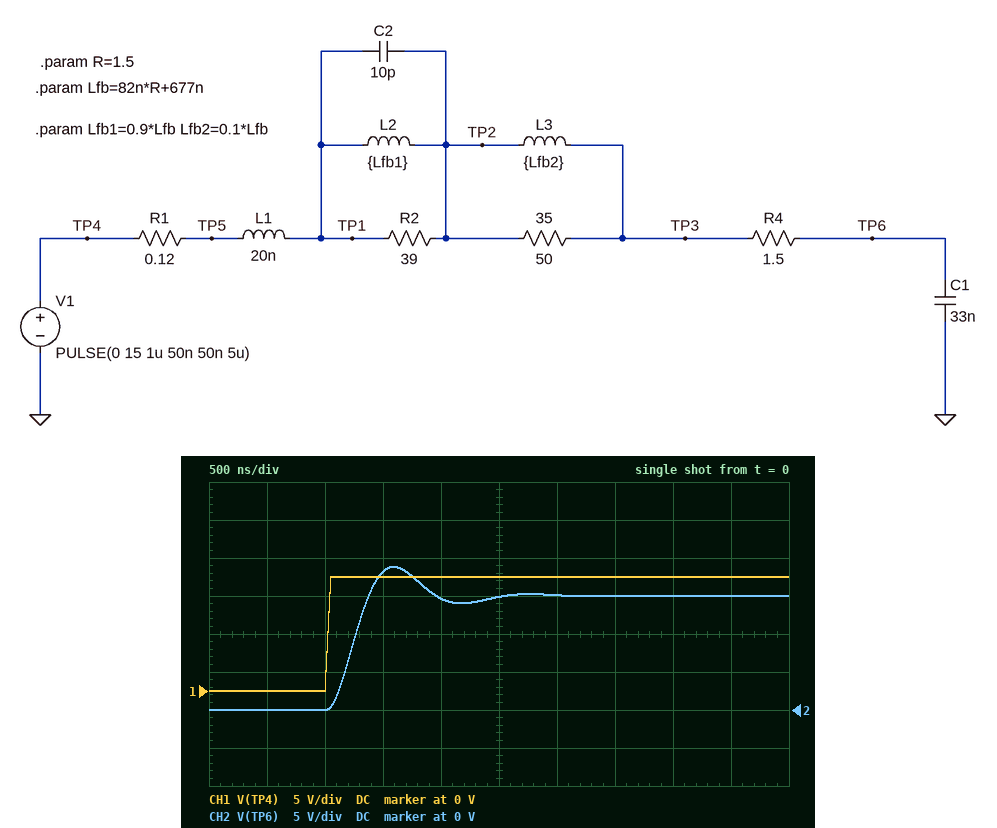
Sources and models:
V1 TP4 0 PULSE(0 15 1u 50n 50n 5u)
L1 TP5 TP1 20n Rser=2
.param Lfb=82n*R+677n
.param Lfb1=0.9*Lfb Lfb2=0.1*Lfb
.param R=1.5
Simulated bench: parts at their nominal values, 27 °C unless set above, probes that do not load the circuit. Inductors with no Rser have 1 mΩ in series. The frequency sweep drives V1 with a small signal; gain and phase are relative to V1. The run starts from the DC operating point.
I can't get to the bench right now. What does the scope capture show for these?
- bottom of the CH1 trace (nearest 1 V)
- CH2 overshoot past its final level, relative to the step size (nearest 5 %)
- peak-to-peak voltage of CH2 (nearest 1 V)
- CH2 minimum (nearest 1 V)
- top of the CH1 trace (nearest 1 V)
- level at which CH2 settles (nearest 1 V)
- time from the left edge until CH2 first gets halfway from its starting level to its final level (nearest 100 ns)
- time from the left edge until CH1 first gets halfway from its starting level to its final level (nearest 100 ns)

0 V
25 %
19 V
0 V
15 V
15 V
1.2 µs
1.0 µs
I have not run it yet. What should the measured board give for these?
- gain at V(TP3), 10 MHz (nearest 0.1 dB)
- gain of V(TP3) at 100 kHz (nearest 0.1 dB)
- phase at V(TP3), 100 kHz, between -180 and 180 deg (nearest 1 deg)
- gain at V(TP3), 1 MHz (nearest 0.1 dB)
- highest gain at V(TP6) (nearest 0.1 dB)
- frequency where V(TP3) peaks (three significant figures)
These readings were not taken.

-27.4 dB
0.1 dB
-3 deg
1.7 dB
2.7 dB
785 kHz
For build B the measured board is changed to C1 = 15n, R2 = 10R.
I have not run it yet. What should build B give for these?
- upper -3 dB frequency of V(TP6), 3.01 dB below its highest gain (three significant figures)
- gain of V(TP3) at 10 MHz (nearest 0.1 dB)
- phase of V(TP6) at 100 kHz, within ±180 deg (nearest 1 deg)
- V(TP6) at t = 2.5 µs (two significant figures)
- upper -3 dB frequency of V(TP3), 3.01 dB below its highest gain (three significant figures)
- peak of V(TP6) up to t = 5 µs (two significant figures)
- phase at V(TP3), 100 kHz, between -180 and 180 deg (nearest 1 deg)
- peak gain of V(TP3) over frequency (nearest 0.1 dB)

1.62 MHz
-18.5 dB
-2 deg
15 V
1.63 MHz
18 V
-1 deg
2.3 dB
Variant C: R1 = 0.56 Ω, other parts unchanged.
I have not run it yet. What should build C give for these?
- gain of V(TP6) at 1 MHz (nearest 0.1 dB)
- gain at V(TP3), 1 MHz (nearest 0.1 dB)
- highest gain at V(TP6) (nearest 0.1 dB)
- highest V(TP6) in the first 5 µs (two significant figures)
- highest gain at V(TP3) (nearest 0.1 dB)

0.4 dB
0.8 dB
2.1 dB
18 V
2.3 dB
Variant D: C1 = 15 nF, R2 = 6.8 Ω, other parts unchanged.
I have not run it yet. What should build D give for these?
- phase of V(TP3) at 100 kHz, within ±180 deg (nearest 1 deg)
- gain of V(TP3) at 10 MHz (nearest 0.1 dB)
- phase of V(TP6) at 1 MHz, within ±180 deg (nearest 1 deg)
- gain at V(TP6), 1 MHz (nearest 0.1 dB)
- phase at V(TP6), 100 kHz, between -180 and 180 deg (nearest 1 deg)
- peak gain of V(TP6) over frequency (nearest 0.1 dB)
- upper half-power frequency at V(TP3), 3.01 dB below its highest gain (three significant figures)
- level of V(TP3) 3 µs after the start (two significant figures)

-1 deg
-16.6 dB
-40 deg
1.5 dB
-2 deg
1.6 dB
1.67 MHz
15 V
